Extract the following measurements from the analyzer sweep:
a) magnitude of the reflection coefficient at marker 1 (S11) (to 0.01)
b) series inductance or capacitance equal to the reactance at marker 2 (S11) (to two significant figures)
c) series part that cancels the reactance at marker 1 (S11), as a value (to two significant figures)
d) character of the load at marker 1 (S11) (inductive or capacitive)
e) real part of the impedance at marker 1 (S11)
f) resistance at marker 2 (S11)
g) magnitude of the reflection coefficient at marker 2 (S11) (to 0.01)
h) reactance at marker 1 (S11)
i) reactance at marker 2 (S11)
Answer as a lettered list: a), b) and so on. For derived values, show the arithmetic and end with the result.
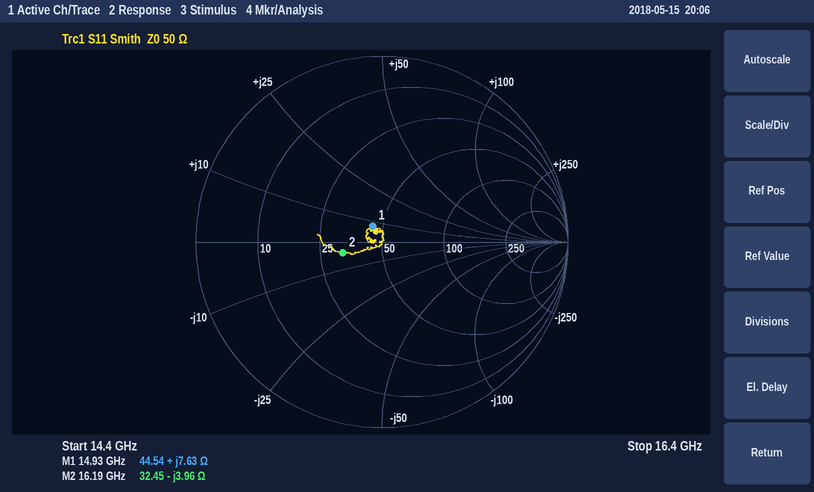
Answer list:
a) 0.10
b) C = 1/(2π × 16.19 GHz × 3.96 Ω) ≈ 2.5 pF
c) C = 1/(2π × 14.93 GHz × 7.63 Ω) ≈ 1.4 pF
d) inductive
e) 44.54 Ω
f) 32.45 Ω
g) 0.22
h) +7.63 Ω
i) -3.96 Ω
